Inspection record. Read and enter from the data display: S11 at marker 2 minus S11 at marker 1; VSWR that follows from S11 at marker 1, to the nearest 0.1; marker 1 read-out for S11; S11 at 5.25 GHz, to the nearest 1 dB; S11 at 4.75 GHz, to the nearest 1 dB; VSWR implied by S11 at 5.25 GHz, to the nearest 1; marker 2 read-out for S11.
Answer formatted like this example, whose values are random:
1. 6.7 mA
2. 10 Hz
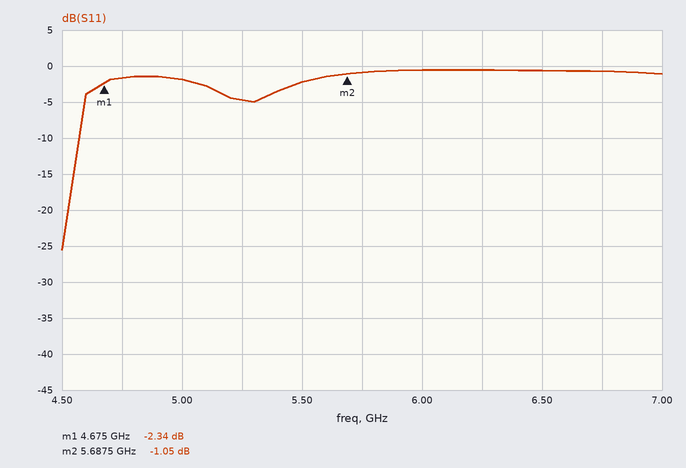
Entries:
1. 1.29 dB
2. 7.5
3. -2.34 dB
4. -5 dB
5. -2 dB
6. 4
7. -1.05 dB
